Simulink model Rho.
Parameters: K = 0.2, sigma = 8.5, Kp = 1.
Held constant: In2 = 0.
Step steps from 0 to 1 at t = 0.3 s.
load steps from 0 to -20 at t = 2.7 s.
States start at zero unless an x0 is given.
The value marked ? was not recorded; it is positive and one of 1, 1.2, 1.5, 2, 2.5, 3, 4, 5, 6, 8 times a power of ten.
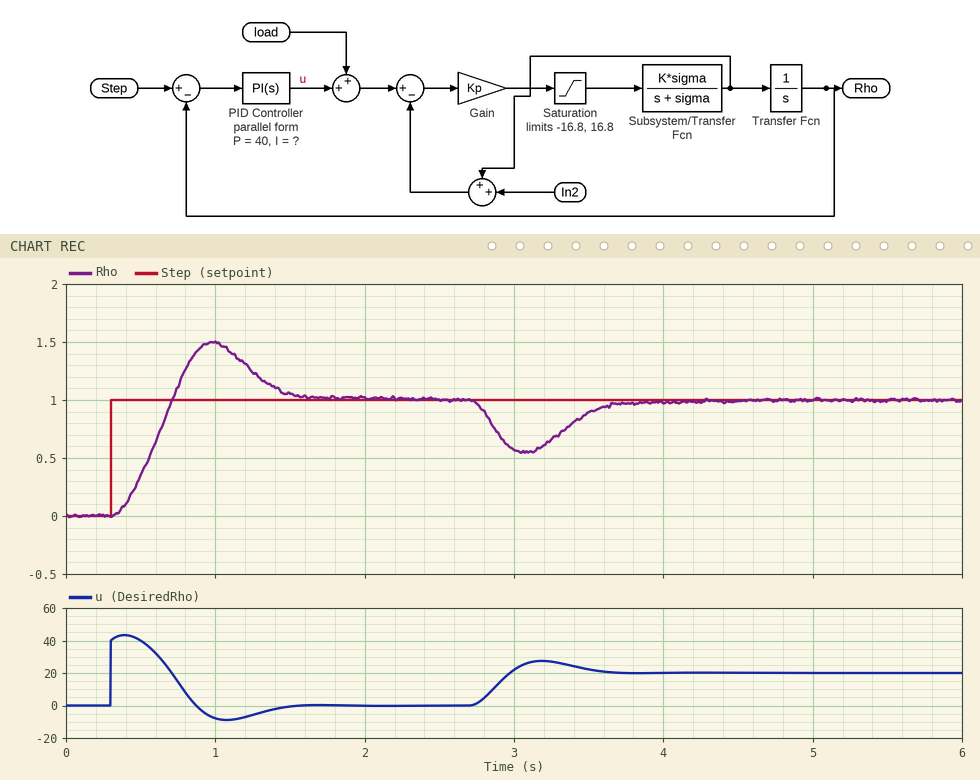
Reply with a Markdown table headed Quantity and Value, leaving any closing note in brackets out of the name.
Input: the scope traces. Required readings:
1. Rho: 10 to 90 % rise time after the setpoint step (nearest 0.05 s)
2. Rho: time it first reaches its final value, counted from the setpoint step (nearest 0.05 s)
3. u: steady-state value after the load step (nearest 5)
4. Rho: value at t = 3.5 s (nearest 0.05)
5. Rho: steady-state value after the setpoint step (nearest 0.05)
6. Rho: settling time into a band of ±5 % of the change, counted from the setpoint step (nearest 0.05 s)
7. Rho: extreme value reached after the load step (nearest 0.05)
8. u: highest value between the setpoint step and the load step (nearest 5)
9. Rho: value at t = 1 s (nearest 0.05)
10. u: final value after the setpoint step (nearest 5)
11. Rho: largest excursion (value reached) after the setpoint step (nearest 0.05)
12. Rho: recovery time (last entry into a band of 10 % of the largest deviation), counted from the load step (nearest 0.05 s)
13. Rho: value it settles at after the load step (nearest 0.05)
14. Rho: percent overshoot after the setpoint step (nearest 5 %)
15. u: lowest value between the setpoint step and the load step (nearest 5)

| Quantity | Value |
|---|---|
| Rho: 10 to 90 % rise time after the setpoint step | 0.30 s |
| Rho: time it first reaches its final value, counted from the setpoint step | 0.40 s |
| u: steady-state value after the load step | 20 |
| Rho: value at t = 3.5 s | 0.90 |
| Rho: steady-state value after the setpoint step | 1.00 |
| Rho: settling time into a band of ±5 % of the change, counted from the setpoint step | 1.20 s |
| Rho: extreme value reached after the load step | 0.55 |
| u: highest value between the setpoint step and the load step | 45 |
| Rho: value at t = 1 s | 1.50 |
| u: final value after the setpoint step | 0 |
| Rho: largest excursion (value reached) after the setpoint step | 1.50 |
| Rho: recovery time (last entry into a band of 10 % of the largest deviation), counted from the load step | 0.95 s |
| Rho: value it settles at after the load step | 1.00 |
| Rho: percent overshoot after the setpoint step | 50 % |
| u: lowest value between the setpoint step and the load step | -10 |
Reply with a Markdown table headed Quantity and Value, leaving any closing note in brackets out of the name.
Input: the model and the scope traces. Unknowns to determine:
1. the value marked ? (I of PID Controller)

| Quantity | Value |
|---|---|
| the value marked ? | 80 |
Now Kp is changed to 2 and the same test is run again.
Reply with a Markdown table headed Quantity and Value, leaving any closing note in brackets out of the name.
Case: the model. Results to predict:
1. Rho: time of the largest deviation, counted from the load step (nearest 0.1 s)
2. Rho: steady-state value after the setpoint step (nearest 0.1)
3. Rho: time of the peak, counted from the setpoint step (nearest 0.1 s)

| Quantity | Value |
|---|---|
| Rho: time of the largest deviation, counted from the load step | 0.3 s |
| Rho: steady-state value after the setpoint step | 1.0 |
| Rho: time of the peak, counted from the setpoint step | 0.6 s |
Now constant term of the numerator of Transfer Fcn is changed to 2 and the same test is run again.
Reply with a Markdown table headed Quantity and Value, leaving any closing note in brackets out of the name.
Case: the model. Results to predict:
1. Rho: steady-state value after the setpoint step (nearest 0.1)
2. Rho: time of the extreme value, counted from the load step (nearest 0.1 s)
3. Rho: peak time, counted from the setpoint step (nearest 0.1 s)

| Quantity | Value |
|---|---|
| Rho: steady-state value after the setpoint step | 1.0 |
| Rho: time of the extreme value, counted from the load step | 0.3 s |
| Rho: peak time, counted from the setpoint step | 0.4 s |
